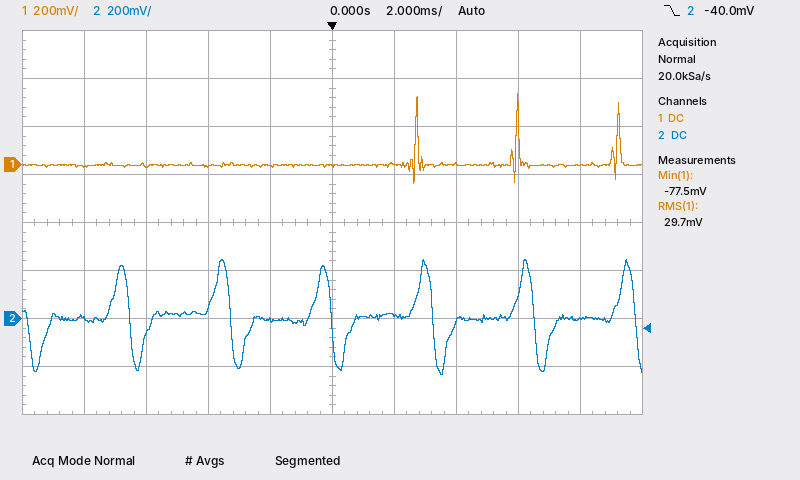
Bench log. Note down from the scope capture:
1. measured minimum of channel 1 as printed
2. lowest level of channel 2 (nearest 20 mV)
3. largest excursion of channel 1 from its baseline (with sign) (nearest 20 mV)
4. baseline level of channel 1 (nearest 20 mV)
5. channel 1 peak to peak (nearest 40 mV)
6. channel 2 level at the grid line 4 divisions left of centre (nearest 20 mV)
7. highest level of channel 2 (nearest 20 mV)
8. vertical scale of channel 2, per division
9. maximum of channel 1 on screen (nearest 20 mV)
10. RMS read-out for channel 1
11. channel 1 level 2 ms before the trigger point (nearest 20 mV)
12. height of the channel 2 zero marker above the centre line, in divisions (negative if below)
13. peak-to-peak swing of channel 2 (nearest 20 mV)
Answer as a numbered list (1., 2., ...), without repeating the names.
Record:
1. -77.5 mV
2. -240 mV
3. +300 mV
4. 0 mV
5. 360 mV
6. 0 mV
7. 240 mV
8. 200 mV
9. 300 mV
10. 29.7 mV
11. 0 mV
12. -2.0 div
13. 480 mV
